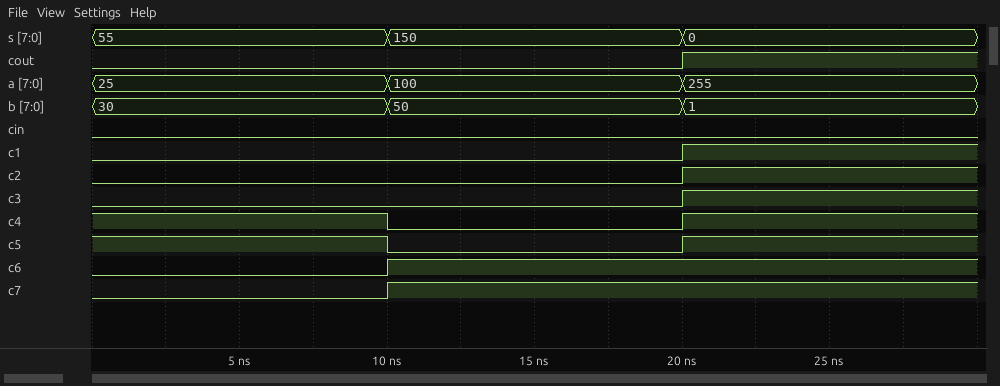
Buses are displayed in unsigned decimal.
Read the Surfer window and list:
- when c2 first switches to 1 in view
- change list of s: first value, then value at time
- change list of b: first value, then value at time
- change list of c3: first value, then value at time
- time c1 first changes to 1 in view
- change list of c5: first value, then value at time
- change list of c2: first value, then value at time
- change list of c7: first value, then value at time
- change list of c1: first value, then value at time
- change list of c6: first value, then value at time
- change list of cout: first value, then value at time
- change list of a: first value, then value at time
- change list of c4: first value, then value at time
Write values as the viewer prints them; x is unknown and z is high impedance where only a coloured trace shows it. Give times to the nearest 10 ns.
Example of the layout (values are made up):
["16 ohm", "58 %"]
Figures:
["20 ns", "55, 150 at 10 ns, 0 at 20 ns", "30, 50 at 10 ns, 1 at 20 ns", "0, 1 at 20 ns", "20 ns", "1, 0 at 10 ns, 1 at 20 ns", "0, 1 at 20 ns", "0, 1 at 10 ns", "0, 1 at 20 ns", "0, 1 at 10 ns", "0, 1 at 20 ns", "25, 100 at 10 ns, 255 at 20 ns", "1, 0 at 10 ns, 1 at 20 ns"]
